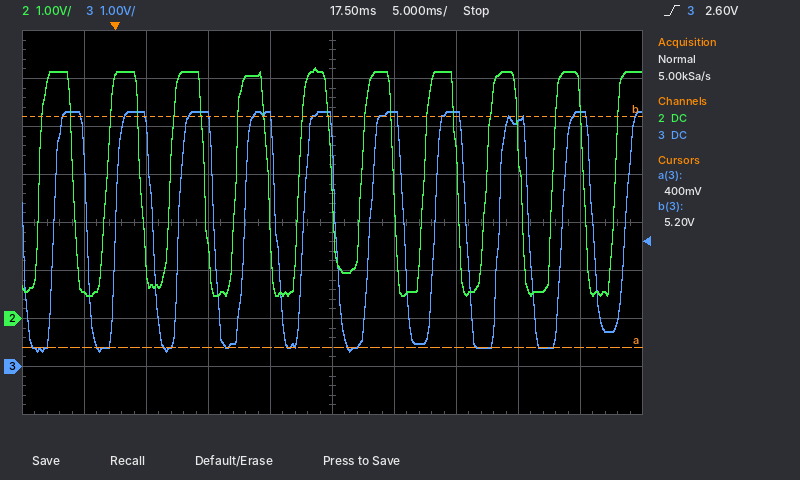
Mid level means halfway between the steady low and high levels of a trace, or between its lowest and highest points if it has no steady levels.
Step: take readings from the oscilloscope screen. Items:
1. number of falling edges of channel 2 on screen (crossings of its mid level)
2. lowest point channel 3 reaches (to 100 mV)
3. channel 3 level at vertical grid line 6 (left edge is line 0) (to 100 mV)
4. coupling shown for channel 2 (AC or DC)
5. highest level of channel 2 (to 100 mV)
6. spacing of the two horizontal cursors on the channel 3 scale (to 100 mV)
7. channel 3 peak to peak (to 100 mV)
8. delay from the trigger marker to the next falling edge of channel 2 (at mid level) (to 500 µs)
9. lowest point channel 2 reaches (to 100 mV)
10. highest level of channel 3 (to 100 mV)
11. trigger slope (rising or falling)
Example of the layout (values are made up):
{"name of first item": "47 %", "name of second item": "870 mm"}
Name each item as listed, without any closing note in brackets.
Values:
{"number of falling edges of channel 2 on screen": "9", "lowest point channel 3 reaches": "300 mV", "channel 3 level at vertical grid line 6 (left edge is line 0)": "5.3 V", "coupling shown for channel 2": "DC", "highest level of channel 2": "5.2 V", "spacing of the two horizontal cursors on the channel 3 scale": "4.8 V", "channel 3 peak to peak": "5.0 V", "delay from the trigger marker to the next falling edge of channel 2 (at mid level)": "2.0 ms", "lowest point channel 2 reaches": "500 mV", "highest level of channel 3": "5.3 V", "trigger slope": "rising"}
